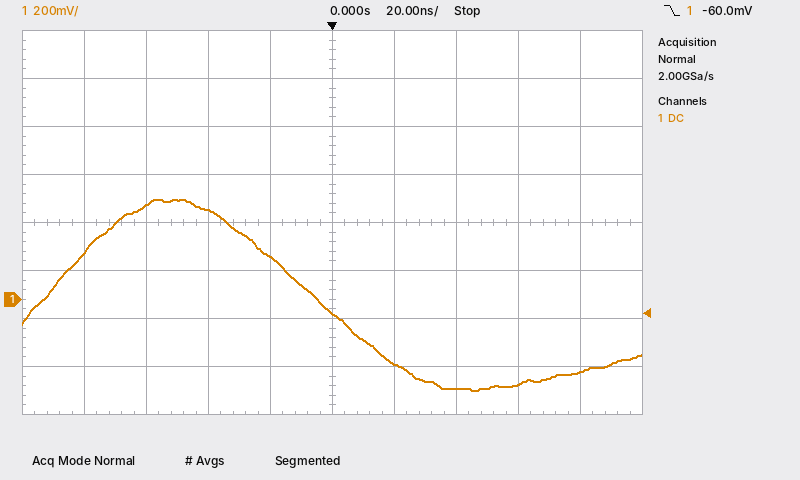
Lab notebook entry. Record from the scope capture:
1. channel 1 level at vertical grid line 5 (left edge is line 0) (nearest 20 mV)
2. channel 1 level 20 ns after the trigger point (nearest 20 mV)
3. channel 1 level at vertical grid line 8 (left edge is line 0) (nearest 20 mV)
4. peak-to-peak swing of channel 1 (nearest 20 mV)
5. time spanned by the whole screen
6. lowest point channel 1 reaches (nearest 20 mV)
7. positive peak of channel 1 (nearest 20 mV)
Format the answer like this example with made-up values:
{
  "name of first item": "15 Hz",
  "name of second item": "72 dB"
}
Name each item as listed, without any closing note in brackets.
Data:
{
  "channel 1 level at vertical grid line 5 (left edge is line 0)": "-60 mV",
  "channel 1 level 20 ns after the trigger point": "-260 mV",
  "channel 1 level at vertical grid line 8 (left edge is line 0)": "-360 mV",
  "peak-to-peak swing of channel 1": "800 mV",
  "time spanned by the whole screen": "200 ns",
  "lowest point channel 1 reaches": "-380 mV",
  "positive peak of channel 1": "420 mV"
}
